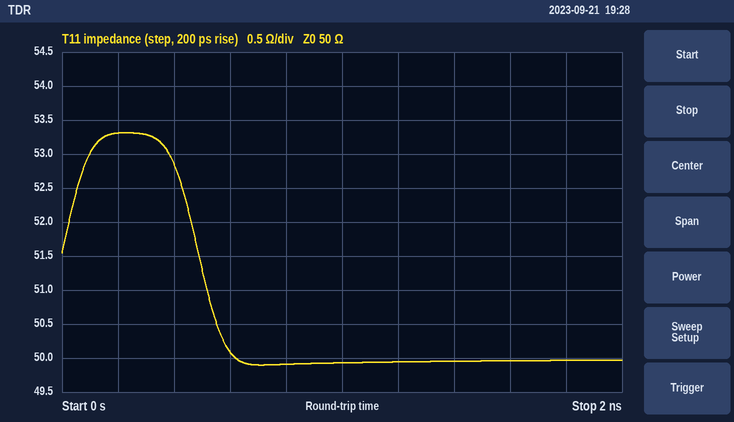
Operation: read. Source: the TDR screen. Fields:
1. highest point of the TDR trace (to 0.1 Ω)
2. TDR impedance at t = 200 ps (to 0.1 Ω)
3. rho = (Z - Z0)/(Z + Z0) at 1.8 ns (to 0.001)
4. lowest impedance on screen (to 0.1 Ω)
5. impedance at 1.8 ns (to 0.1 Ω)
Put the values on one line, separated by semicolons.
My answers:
53.3 Ω; 53.3 Ω; 0.000; 49.9 Ω; 50.0 Ω
